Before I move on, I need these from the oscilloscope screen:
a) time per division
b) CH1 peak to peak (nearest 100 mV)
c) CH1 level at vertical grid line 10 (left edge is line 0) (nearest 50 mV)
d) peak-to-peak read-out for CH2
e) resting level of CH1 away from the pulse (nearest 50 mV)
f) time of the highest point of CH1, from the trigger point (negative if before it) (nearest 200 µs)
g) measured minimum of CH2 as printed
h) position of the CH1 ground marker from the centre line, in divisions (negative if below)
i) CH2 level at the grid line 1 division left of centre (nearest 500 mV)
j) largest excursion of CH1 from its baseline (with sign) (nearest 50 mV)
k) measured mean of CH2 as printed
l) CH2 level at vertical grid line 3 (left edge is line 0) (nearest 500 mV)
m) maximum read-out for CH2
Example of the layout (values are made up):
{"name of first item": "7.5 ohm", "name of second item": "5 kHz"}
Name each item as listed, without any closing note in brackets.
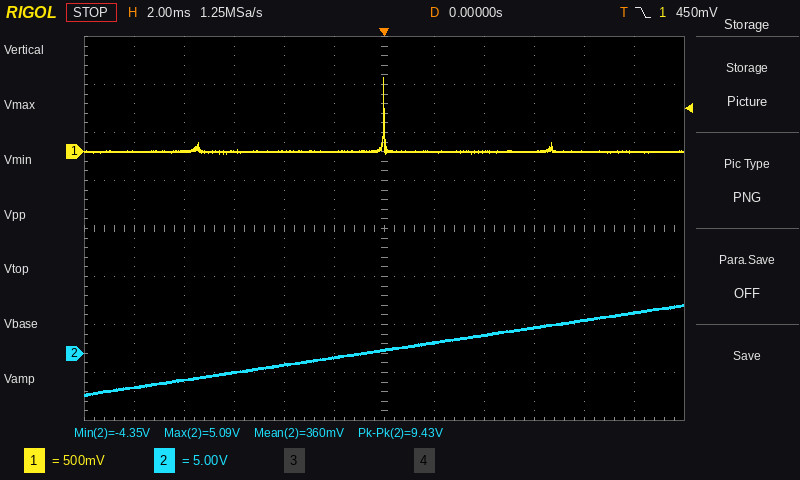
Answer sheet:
{"time per division": "2 ms", "CH1 peak to peak": "800 mV", "CH1 level at vertical grid line 10 (left edge is line 0)": "0 mV", "peak-to-peak read-out for CH2": "9.43 V", "resting level of CH1 away from the pulse": "0 mV", "time of the highest point of CH1, from the trigger point (negative if before it)": "0.0 ms", "measured minimum of CH2 as printed": "-4.35 V", "position of the CH1 ground marker from the centre line, in divisions": "+1.6 div", "CH2 level at the grid line 1 division left of centre": "-500 mV", "largest excursion of CH1 from its baseline (with sign)": "+750 mV", "measured mean of CH2 as printed": "360 mV", "CH2 level at vertical grid line 3 (left edge is line 0)": "-2.0 V", "maximum read-out for CH2": "5.09 V"}
